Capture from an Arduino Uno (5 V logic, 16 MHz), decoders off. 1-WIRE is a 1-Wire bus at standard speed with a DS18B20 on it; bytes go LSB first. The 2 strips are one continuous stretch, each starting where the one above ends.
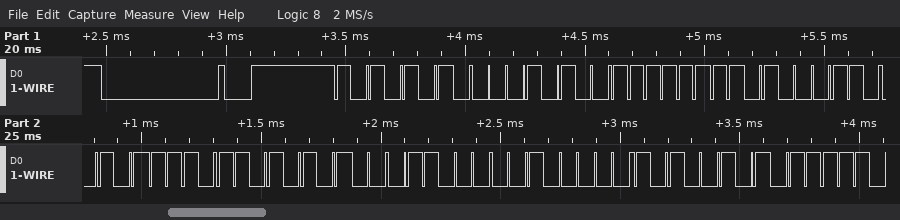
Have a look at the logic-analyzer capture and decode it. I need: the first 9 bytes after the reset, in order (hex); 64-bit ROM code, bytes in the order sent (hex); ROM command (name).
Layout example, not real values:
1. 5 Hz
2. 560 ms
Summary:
1. 55 28 FF 62 7A AB 18 04 A5
2. 28 FF 62 7A AB 18 04 A5
3. Match ROM
